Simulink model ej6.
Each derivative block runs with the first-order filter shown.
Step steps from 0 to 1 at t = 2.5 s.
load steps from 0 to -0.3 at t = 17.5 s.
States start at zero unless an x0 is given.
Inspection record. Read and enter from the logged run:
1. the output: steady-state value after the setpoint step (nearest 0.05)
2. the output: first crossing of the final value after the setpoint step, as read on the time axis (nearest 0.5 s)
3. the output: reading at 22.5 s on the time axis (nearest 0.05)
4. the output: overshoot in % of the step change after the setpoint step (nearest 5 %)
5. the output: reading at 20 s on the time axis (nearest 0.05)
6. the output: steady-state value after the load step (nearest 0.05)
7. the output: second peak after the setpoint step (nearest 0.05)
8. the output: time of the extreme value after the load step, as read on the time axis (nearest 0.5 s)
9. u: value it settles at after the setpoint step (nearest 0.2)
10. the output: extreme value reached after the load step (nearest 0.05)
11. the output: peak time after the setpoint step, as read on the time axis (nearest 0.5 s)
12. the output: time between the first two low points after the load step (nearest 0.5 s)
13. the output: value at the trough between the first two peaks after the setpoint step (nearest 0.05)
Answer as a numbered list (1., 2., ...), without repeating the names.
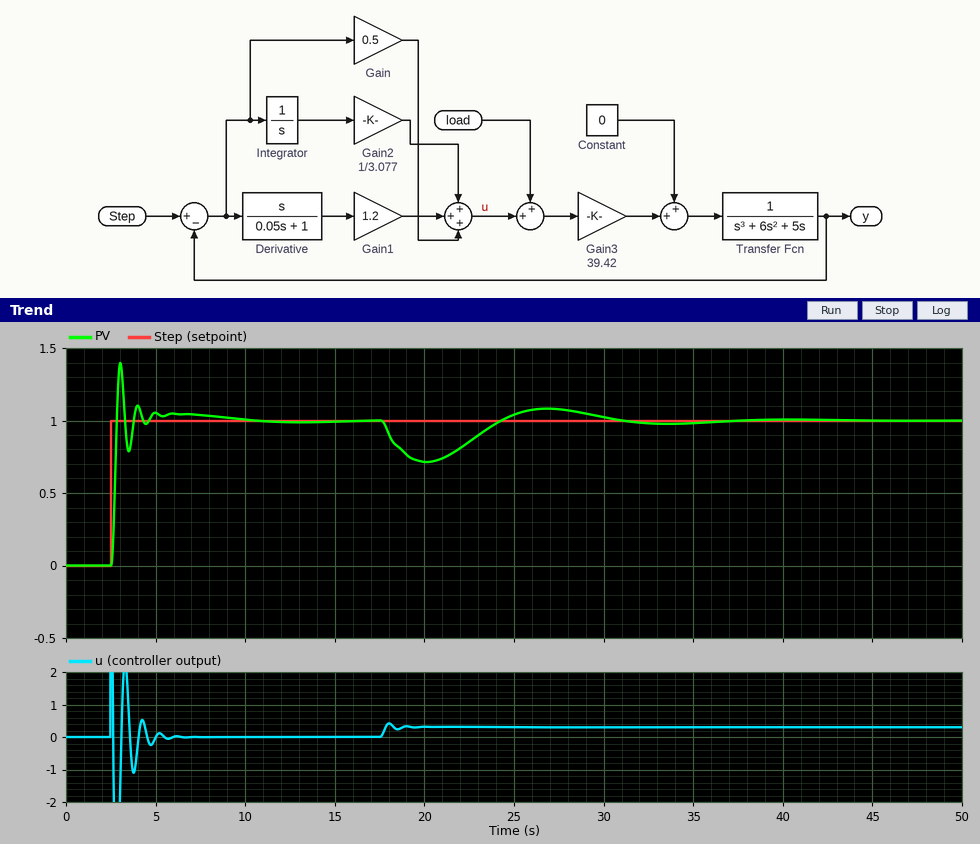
1. 1.00
2. 3.0 s
3. 0.85
4. 40 %
5. 0.70
6. 1.00
7. 1.10
8. 20.0 s
9. 0.0
10. 0.70
11. 3.0 s
12. 13.5 s
13. 0.80
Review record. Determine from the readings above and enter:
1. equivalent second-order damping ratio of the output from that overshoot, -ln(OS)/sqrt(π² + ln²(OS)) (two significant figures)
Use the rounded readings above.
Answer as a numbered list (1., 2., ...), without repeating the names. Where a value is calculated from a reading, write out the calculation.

1. ln(0.4) = -0.916; 0.916 / sqrt(9.870 + 0.840) = 0.28
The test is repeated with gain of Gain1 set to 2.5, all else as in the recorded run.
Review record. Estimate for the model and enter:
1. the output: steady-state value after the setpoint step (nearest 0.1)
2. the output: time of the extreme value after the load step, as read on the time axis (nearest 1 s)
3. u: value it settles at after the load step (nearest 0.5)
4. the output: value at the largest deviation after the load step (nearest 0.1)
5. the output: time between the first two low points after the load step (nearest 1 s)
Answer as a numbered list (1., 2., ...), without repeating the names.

1. 1.0
2. 21 s
3. 0.5
4. 0.8
5. 18 s
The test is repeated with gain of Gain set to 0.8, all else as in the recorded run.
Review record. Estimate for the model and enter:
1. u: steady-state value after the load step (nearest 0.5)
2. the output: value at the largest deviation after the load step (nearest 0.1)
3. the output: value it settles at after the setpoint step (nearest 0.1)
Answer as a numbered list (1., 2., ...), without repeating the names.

1. 0.5
2. 0.8
3. 1.0
